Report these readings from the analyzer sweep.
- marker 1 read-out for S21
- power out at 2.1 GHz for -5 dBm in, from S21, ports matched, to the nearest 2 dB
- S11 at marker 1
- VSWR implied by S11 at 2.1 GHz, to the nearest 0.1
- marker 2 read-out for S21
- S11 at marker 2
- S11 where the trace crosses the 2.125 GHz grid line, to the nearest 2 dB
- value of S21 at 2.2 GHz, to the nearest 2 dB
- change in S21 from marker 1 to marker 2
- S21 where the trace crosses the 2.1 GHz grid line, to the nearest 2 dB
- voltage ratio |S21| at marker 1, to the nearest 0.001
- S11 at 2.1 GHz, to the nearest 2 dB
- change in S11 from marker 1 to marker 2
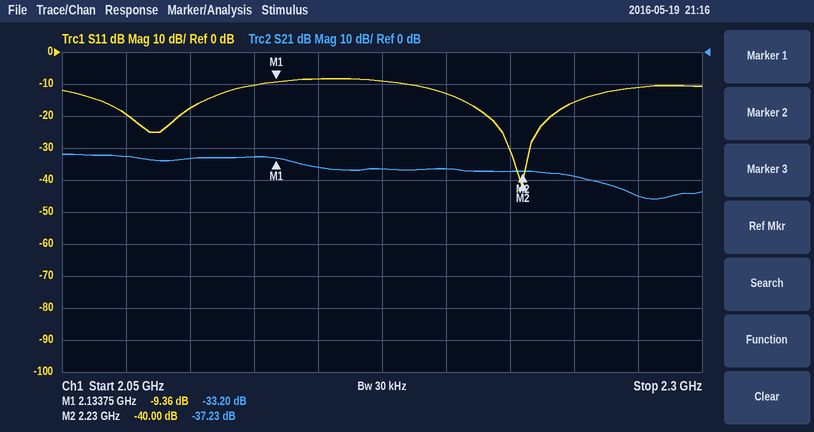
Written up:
-33.20 dB
-38 dBm
-9.36 dB
1.3
-37.23 dB
-40.00 dB
-10 dB
-36 dB
-4.03 dB
-34 dB
0.022
-18 dB
-30.64 dB
